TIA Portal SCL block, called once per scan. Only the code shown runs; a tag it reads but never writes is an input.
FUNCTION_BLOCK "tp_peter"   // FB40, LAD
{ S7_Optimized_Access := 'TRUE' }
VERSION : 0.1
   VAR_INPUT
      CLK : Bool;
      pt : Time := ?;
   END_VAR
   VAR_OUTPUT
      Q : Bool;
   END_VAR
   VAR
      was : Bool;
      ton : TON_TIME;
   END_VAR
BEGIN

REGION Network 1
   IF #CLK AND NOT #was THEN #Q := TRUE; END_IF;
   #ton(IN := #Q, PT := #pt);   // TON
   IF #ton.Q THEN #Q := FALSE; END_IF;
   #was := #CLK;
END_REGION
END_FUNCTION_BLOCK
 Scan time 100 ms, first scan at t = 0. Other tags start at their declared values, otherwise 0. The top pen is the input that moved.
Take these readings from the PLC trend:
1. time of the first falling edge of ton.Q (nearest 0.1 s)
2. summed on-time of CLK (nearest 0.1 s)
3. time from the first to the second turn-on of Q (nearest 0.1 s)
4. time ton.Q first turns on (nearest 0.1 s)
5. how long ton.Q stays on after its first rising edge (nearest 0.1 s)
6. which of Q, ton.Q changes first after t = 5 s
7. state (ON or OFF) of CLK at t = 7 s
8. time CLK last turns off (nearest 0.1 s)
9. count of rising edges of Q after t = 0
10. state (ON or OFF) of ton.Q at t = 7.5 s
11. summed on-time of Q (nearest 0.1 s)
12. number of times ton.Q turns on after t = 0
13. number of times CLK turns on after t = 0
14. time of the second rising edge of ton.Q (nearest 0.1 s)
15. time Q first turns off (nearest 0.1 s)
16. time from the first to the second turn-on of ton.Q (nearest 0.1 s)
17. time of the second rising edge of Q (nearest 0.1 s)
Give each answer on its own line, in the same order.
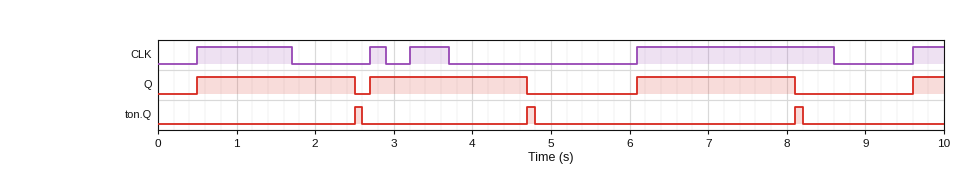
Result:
2.6 s
4.8 s
2.2 s
2.5 s
0.1 s
Q
ON
8.6 s
4
OFF
6.4 s
3
5
4.7 s
2.5 s
2.2 s
2.7 s
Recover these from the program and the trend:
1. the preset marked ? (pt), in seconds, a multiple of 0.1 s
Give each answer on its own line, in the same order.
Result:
2.0 s
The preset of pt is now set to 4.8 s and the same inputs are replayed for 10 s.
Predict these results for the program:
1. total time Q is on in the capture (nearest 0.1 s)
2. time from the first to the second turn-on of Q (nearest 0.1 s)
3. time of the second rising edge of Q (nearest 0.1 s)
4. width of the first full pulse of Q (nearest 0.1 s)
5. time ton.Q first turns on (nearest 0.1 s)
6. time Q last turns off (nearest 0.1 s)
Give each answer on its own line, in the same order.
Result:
8.7 s
5.6 s
6.1 s
4.8 s
5.3 s
5.3 s
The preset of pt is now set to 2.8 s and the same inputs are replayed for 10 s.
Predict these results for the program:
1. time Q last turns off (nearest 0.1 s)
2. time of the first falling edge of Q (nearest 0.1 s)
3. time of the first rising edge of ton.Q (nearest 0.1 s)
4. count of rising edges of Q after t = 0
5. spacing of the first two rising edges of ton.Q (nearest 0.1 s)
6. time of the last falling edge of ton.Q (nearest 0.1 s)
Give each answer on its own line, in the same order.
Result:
8.9 s
3.3 s
3.3 s
3
5.6 s
9.0 s
